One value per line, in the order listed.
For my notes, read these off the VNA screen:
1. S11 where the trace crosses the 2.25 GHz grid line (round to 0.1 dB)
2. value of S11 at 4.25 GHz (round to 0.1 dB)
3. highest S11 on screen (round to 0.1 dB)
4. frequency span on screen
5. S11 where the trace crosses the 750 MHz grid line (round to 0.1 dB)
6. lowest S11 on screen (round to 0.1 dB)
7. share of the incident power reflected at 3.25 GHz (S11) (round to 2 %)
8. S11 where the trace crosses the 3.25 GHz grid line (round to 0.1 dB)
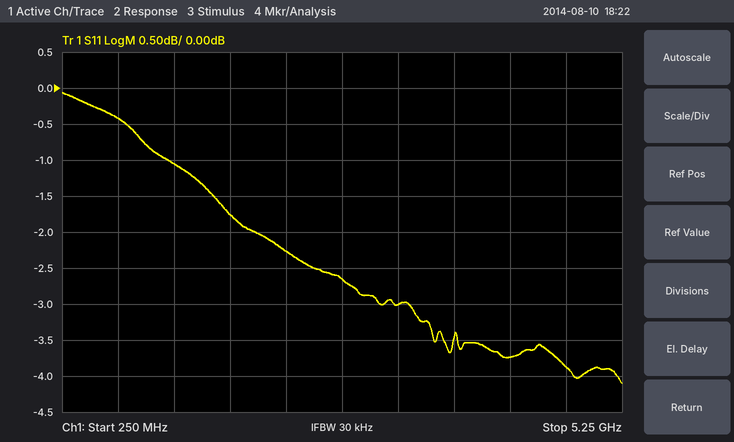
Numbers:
-2.3 dB
-3.7 dB
-0.1 dB
5 GHz
-0.4 dB
-4.1 dB
50 %
-3.0 dB
